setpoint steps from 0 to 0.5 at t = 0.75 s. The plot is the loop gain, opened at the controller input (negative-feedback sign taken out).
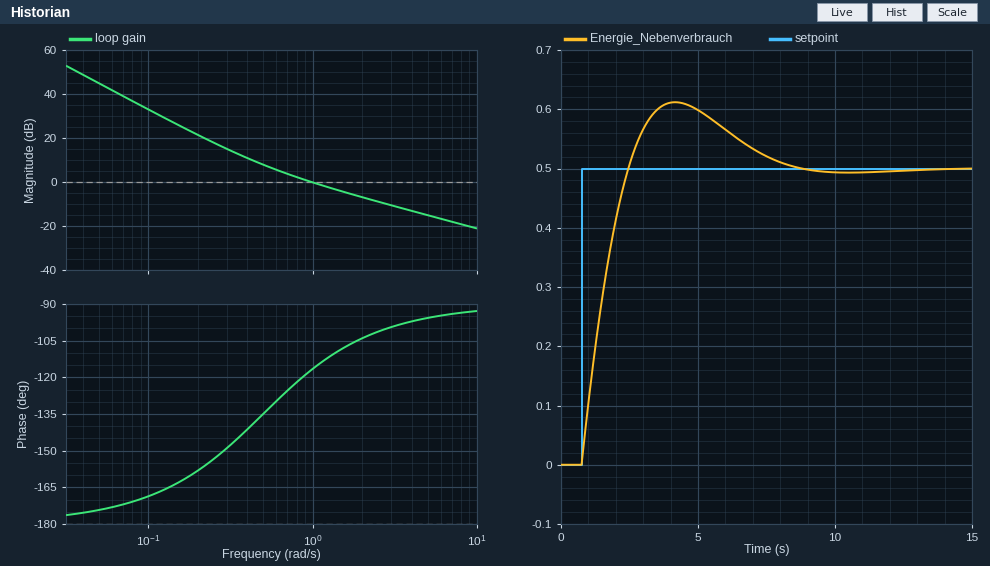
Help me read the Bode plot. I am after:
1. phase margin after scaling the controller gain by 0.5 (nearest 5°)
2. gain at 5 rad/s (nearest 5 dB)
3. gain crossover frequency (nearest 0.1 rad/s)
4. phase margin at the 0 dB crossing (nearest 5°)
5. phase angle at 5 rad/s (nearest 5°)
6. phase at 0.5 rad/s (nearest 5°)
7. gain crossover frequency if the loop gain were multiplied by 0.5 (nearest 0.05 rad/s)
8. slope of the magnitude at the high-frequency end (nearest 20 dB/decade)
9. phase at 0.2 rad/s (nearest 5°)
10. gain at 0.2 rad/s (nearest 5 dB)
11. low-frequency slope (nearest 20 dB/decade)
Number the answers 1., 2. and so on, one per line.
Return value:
1. 50°
2. -15 dB
3. 1.0 rad/s
4. 65°
5. -95°
6. -135°
7. 0.60 rad/s
8. -20 dB/decade
9. -160°
10. 20 dB
11. -40 dB/decade
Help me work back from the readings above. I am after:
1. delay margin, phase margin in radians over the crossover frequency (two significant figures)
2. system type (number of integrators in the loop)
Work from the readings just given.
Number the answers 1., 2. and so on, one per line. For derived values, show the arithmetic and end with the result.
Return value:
1. 65 × π / 180 / 1 = 1.1 s
2. 2
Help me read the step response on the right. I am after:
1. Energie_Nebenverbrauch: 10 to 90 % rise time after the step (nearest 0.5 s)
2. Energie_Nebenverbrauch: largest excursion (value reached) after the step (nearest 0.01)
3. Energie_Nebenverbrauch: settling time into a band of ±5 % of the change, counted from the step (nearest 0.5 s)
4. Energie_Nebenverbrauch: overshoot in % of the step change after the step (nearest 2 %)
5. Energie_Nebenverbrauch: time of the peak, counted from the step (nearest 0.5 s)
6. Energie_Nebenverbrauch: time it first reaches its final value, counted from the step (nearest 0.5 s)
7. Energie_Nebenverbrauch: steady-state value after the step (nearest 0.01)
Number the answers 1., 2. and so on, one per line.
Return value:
1. 1.5 s
2. 0.61
3. 6.5 s
4. 22 %
5. 3.5 s
6. 1.5 s
7. 0.50
